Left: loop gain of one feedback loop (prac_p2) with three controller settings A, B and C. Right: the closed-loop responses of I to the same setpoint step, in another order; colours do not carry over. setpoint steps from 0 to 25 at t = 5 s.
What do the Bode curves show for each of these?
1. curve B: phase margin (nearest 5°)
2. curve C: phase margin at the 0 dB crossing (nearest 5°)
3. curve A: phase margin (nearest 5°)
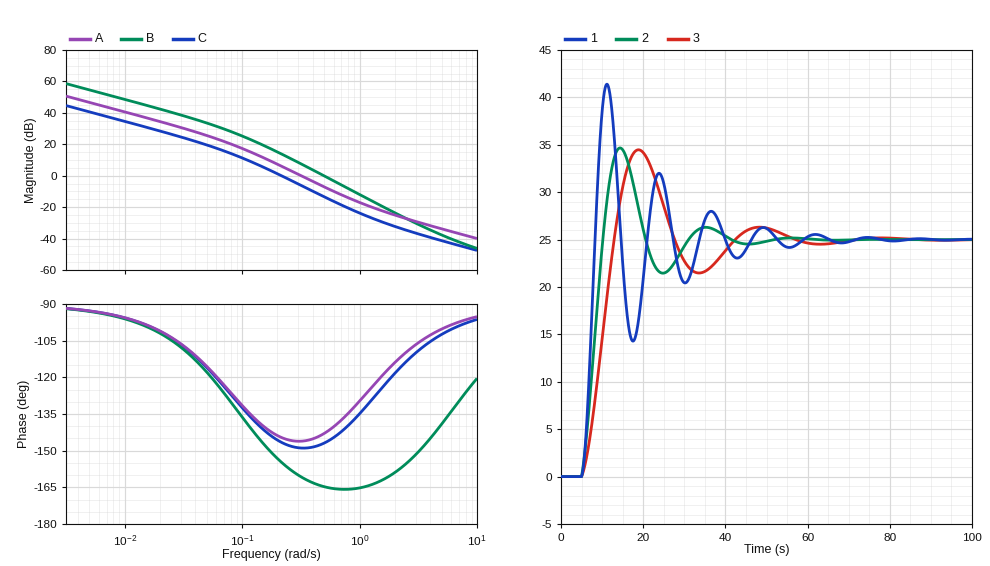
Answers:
15°
35°
35°
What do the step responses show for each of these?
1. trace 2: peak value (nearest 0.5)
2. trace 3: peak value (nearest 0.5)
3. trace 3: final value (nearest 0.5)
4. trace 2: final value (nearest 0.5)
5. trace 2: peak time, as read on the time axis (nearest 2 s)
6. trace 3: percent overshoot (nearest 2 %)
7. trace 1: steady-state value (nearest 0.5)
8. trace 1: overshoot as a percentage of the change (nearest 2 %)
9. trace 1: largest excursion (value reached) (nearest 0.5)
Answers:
34.5
34.5
25.0
25.0
14 s
38 %
25.0
66 %
41.5
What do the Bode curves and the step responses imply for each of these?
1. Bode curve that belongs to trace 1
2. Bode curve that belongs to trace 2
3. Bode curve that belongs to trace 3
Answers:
B
A
C
